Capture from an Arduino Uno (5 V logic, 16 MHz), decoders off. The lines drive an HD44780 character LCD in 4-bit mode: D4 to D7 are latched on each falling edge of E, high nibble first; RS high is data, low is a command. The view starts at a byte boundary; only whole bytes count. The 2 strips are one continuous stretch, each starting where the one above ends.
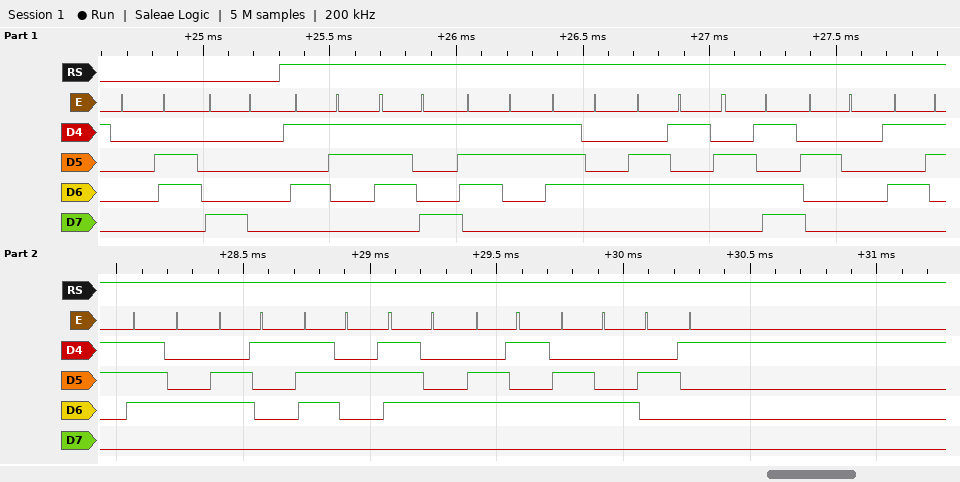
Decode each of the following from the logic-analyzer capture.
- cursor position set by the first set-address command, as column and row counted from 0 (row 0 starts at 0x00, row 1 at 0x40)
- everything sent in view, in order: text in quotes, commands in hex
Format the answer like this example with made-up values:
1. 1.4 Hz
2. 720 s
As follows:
1. column 0, row 0
2. 0x06 0x80 "System Started!"
